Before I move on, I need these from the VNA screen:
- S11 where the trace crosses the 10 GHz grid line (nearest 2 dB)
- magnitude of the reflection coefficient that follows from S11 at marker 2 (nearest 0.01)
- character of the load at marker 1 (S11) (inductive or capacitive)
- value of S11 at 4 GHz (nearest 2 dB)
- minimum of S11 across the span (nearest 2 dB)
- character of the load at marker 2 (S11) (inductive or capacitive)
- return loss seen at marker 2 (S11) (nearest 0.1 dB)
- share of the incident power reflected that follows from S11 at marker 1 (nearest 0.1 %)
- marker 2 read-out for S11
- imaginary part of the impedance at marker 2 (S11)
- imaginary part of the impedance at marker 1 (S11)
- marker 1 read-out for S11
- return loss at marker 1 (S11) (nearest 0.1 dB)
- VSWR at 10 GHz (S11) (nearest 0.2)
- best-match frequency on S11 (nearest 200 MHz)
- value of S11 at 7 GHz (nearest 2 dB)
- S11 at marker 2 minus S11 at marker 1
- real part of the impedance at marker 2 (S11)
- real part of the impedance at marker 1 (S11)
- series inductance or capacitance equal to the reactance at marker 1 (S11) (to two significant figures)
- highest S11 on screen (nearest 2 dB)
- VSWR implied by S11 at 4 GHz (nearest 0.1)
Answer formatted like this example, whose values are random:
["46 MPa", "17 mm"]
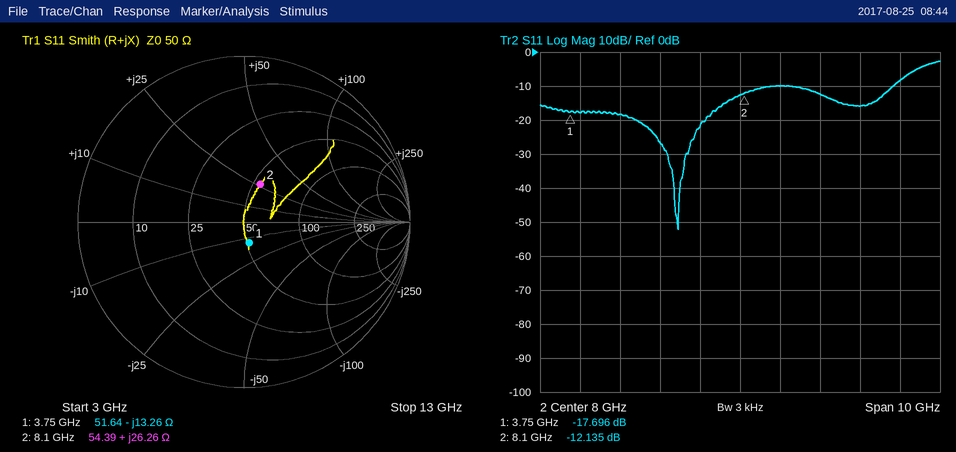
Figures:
["-12 dB", "0.25", "capacitive", "-18 dB", "-52 dB", "inductive", "12.1 dB", "1.7 %", "-12.135 dB", "+26.26 Ω", "-13.26 Ω", "-17.696 dB", "17.7 dB", "1.6", "6.4 GHz", "-22 dB", "5.561 dB", "54.39 Ω", "51.64 Ω", "3.2 pF", "-2 dB", "1.3"]
